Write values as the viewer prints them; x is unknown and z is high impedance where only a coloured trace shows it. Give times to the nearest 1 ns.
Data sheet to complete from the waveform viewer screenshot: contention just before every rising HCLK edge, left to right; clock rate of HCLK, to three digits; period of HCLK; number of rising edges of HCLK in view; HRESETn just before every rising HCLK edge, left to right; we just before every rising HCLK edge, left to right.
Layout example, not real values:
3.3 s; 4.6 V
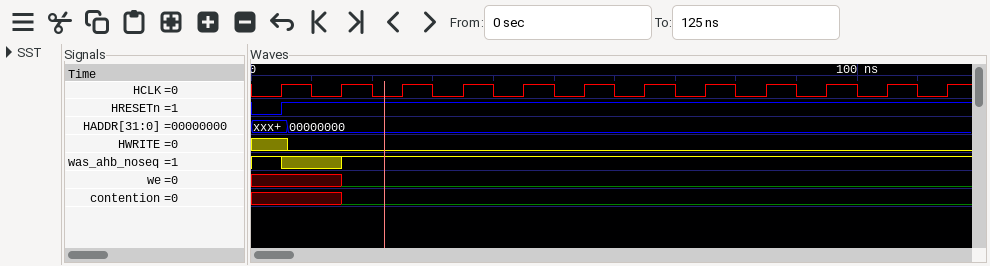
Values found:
x x 0 0 0 0 0 0 0 0 0 0; 100 MHz; 10 ns; 12; 0 1 1 1 1 1 1 1 1 1 1 1; x x 0 0 0 0 0 0 0 0 0 0
